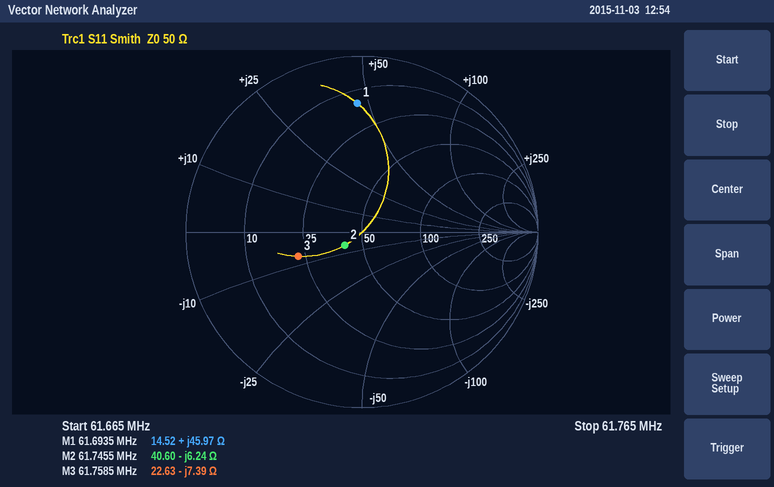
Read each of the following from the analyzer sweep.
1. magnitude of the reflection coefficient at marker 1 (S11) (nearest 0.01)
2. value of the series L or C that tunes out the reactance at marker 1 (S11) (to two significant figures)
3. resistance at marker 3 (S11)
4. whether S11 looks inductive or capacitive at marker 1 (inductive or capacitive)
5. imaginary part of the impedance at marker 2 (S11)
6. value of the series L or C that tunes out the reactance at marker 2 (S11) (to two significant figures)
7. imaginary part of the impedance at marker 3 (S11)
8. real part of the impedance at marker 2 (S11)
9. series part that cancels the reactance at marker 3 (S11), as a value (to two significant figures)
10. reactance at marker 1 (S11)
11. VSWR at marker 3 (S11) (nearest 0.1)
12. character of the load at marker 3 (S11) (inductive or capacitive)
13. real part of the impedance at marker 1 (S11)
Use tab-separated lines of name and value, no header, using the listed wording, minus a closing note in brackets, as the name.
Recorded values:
magnitude of the reflection coefficient at marker 1 (S11)	0.73
value of the series L or C that tunes out the reactance at marker 1 (S11)	56 pF
resistance at marker 3	22.63 Ω
whether S11 looks inductive or capacitive at marker 1	inductive
imaginary part of the impedance at marker 2	-6.24 Ω
value of the series L or C that tunes out the reactance at marker 2 (S11)	16 nH
imaginary part of the impedance at marker 3	-7.39 Ω
real part of the impedance at marker 2	40.60 Ω
series part that cancels the reactance at marker 3 (S11), as a value	19 nH
reactance at marker 1	+45.97 Ω
VSWR at marker 3 (S11)	2.3
character of the load at marker 3 (S11)	capacitive
real part of the impedance at marker 1	14.52 Ω
